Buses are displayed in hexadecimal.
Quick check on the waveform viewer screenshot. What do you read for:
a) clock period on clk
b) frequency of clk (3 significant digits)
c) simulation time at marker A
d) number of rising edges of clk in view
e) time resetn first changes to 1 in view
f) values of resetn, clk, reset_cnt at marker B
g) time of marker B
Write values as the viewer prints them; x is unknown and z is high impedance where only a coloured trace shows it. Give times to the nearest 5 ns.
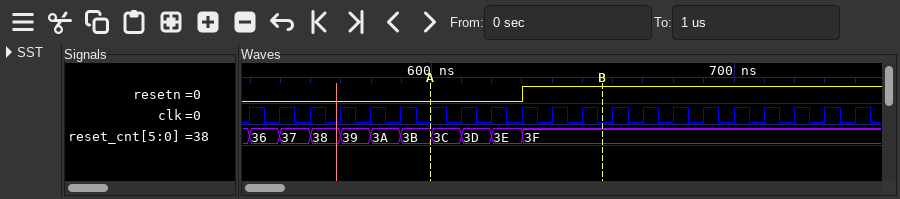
10 ns
100 MHz
600 ns
21
630 ns
resetn=1, clk=0, reset_cnt=3F
655 ns
